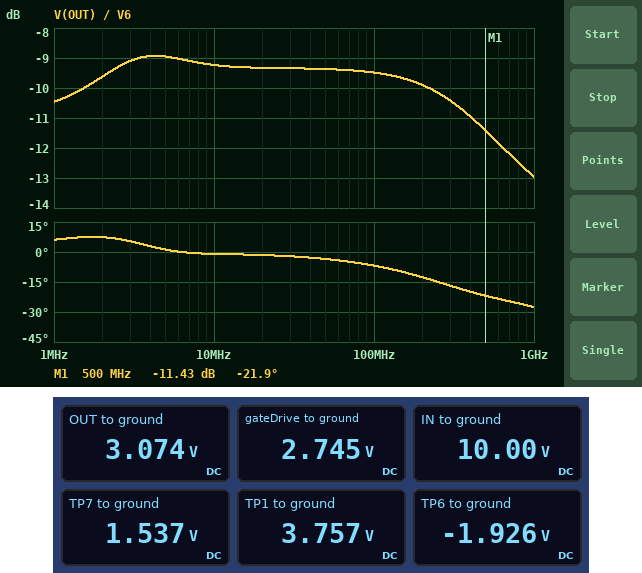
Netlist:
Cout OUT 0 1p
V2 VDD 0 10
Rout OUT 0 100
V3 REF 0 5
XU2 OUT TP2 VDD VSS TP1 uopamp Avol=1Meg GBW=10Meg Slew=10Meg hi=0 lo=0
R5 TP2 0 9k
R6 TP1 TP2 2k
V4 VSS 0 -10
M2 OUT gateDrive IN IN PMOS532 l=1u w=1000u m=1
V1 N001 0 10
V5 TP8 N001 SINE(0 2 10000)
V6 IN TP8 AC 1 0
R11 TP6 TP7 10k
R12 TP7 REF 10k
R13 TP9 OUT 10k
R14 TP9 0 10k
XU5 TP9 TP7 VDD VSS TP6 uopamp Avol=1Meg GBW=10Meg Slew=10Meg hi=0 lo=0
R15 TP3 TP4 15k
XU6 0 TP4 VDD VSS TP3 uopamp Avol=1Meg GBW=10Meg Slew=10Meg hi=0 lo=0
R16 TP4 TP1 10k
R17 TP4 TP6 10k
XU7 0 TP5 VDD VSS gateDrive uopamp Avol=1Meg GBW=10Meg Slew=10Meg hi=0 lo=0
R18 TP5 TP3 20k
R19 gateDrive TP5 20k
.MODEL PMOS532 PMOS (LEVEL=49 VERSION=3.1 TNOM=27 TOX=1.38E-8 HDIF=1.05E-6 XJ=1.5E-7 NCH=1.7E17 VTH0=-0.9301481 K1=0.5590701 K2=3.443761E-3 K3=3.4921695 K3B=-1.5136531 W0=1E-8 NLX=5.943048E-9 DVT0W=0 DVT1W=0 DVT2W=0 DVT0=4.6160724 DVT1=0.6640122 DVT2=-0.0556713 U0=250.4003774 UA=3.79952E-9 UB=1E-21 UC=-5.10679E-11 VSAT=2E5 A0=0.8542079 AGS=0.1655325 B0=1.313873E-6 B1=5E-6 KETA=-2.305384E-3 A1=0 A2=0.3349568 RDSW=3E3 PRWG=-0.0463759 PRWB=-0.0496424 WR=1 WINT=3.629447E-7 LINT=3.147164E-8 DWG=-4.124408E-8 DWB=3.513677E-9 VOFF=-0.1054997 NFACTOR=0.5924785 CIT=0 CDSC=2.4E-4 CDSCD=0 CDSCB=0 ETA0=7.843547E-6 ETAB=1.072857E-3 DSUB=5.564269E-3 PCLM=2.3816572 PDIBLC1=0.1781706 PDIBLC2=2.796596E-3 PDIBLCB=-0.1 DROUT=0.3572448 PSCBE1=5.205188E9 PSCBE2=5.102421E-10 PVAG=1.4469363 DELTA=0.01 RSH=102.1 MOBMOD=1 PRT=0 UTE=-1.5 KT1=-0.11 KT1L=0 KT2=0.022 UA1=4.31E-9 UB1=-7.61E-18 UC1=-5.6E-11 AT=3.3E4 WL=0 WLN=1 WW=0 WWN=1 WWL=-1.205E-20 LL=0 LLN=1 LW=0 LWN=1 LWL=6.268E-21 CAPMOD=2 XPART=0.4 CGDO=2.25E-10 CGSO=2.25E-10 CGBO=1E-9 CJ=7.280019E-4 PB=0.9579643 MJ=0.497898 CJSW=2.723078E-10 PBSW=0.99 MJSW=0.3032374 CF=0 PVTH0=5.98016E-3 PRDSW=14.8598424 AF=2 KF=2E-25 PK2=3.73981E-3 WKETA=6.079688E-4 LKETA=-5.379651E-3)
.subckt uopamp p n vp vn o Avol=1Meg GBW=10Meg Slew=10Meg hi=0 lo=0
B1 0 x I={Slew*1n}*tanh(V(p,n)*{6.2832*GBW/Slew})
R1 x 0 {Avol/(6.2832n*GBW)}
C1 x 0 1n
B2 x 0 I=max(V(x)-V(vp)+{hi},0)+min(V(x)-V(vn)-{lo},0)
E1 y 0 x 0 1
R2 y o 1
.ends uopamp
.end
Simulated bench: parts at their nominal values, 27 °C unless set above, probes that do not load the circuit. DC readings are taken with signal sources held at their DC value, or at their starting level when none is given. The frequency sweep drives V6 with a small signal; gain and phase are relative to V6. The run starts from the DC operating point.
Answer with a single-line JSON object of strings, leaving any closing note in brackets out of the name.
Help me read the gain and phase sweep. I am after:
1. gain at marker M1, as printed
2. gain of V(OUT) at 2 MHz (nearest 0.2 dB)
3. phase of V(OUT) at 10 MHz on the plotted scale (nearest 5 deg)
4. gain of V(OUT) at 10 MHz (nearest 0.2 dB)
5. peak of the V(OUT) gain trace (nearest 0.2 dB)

{"gain at marker M1, as printed": "-11.43 dB", "gain of V(OUT) at 2 MHz": "-9.6 dB", "phase of V(OUT) at 10 MHz on the plotted scale": "0 deg", "gain of V(OUT) at 10 MHz": "-9.2 dB", "peak of the V(OUT) gain trace": "-9.0 dB"}
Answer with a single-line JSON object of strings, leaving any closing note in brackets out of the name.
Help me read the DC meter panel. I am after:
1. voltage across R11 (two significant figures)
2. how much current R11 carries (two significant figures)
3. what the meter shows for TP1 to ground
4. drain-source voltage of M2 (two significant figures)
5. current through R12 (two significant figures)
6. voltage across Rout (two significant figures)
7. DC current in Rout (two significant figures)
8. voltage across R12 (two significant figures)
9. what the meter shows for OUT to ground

{"voltage across R11": "3.5 V", "how much current R11 carries": "350 µA", "what the meter shows for TP1 to ground": "3.757 V", "drain-source voltage of M2": "-6.9 V", "current through R12": "350 µA", "voltage across Rout": "3.1 V", "DC current in Rout": "31 mA", "voltage across R12": "3.5 V", "what the meter shows for OUT to ground": "3.074 V"}
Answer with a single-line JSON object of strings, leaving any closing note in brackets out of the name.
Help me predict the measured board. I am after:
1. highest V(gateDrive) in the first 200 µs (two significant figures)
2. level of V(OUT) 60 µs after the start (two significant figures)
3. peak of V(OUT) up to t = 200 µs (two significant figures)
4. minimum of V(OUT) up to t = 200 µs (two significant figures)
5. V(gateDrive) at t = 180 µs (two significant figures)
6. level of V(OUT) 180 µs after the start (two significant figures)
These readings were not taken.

{"highest V(gateDrive) in the first 200 µs": "4.6 V", "level of V(OUT) 60 µs after the start": "2.7 V", "peak of V(OUT) up to t = 200 µs": "3.6 V", "minimum of V(OUT) up to t = 200 µs": "2.5 V", "V(gateDrive) at t = 180 µs": "890 mV", "level of V(OUT) 180 µs after the start": "2.5 V"}
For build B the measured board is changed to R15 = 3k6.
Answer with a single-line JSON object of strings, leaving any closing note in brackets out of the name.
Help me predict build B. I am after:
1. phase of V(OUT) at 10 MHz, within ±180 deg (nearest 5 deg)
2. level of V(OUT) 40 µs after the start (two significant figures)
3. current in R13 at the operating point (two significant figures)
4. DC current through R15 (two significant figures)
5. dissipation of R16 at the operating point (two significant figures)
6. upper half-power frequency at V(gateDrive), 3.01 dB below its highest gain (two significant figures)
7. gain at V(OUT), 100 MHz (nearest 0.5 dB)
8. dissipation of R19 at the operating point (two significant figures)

{"phase of V(OUT) at 10 MHz, within ±180 deg": "0 deg", "level of V(OUT) 40 µs after the start": "3.5 V", "current in R13 at the operating point": "160 µA", "DC current through R15": "200 µA", "dissipation of R16 at the operating point": "1.5 mW", "upper half-power frequency at V(gateDrive), 3.01 dB below its highest gain": "2.9 MHz", "gain at V(OUT), 100 MHz": "-10.0 dB", "dissipation of R19 at the operating point": "25 µW"}
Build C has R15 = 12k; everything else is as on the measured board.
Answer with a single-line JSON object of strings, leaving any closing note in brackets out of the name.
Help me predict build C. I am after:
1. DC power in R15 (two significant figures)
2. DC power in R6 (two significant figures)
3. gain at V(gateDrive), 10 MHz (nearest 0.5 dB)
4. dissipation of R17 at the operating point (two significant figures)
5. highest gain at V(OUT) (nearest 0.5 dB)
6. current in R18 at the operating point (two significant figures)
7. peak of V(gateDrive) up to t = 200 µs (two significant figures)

{"DC power in R15": "430 µW", "DC power in R6": "240 µW", "gain at V(gateDrive), 10 MHz": "-24.0 dB", "dissipation of R17 at the operating point": "360 µW", "highest gain at V(OUT)": "-9.5 dB", "current in R18 at the operating point": "110 µA", "peak of V(gateDrive) up to t = 200 µs": "3.8 V"}
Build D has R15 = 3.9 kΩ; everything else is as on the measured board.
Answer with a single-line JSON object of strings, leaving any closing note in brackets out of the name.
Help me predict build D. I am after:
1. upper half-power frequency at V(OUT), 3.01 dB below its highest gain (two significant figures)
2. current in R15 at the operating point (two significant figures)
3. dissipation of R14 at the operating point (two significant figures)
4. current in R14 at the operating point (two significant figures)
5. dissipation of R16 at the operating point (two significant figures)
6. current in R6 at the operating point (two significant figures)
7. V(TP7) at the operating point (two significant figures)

{"upper half-power frequency at V(OUT), 3.01 dB below its highest gain": "820 MHz", "current in R15 at the operating point": "200 µA", "dissipation of R14 at the operating point": "250 µW", "current in R14 at the operating point": "160 µA", "dissipation of R16 at the operating point": "1.5 mW", "current in R6 at the operating point": "350 µA", "V(TP7) at the operating point": "1.6 V"}
